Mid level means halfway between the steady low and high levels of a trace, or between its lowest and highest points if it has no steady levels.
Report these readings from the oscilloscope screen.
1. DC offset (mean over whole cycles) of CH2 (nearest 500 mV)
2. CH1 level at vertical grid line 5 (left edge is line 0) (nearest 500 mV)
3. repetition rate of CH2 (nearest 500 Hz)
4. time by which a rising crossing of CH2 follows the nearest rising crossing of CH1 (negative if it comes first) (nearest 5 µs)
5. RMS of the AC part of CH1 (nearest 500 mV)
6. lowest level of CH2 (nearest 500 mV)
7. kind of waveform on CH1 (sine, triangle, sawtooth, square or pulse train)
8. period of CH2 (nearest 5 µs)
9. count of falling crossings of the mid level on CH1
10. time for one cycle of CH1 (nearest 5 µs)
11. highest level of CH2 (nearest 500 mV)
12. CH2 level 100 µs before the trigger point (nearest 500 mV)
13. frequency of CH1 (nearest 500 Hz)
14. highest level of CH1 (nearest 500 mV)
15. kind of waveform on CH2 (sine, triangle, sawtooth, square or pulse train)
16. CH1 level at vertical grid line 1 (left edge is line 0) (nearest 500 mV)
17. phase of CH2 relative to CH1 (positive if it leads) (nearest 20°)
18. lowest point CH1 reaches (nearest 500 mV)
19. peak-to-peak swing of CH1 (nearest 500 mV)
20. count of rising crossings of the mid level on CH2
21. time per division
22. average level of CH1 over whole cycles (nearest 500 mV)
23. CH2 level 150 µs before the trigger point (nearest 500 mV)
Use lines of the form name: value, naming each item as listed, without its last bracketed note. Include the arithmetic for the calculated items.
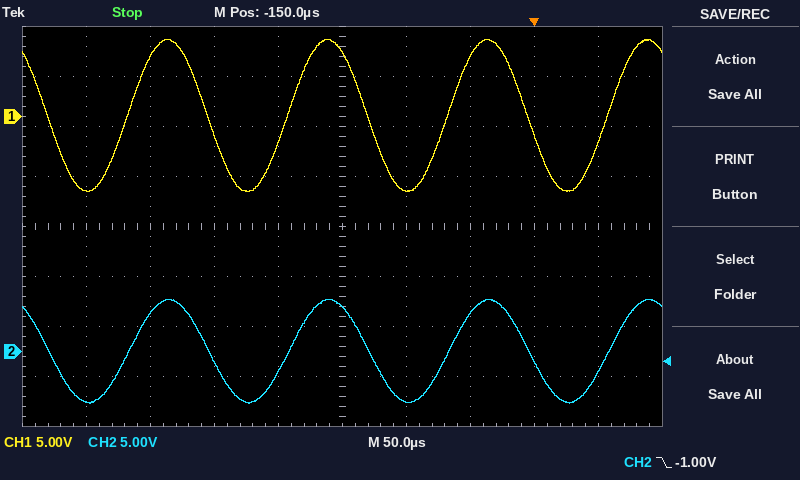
DC offset (mean over whole cycles) of CH2: (5.0 V + (-5.0 V)) / 2 ≈ 0.0 V
CH1 level at vertical grid line 5 (left edge is line 0): 6.5 V
repetition rate of CH2: 1 / 125 µs ≈ 8.0 kHz
time by which a rising crossing of CH2 follows the nearest rising crossing of CH1 (negative if it comes first): 0 µs
RMS of the AC part of CH1: 15.0 V / (2√2) ≈ 5.30 V, so 5.5 V to the nearest 500 mV
lowest level of CH2: -5.0 V
kind of waveform on CH1: sine
period of CH2: 125 µs
count of falling crossings of the mid level on CH1: 4
time for one cycle of CH1: 125 µs
highest level of CH2: 5.0 V
CH2 level 100 µs before the trigger point: -5.0 V
frequency of CH1: 1 / 125 µs ≈ 8.0 kHz
highest level of CH1: 7.5 V
kind of waveform on CH2: sine
CH1 level at vertical grid line 1 (left edge is line 0): -7.5 V
phase of CH2 relative to CH1 (positive if it leads): −360° × (0 µs) / 125 µs ≈ 0°
lowest point CH1 reaches: -7.5 V
peak-to-peak swing of CH1: 7.5 V − (-7.5 V) = 15.0 V
count of rising crossings of the mid level on CH2: 4
time per division: 50 µs
average level of CH1 over whole cycles: (7.5 V + (-7.5 V)) / 2 ≈ 0.0 V
CH2 level 150 µs before the trigger point: 4.5 V
